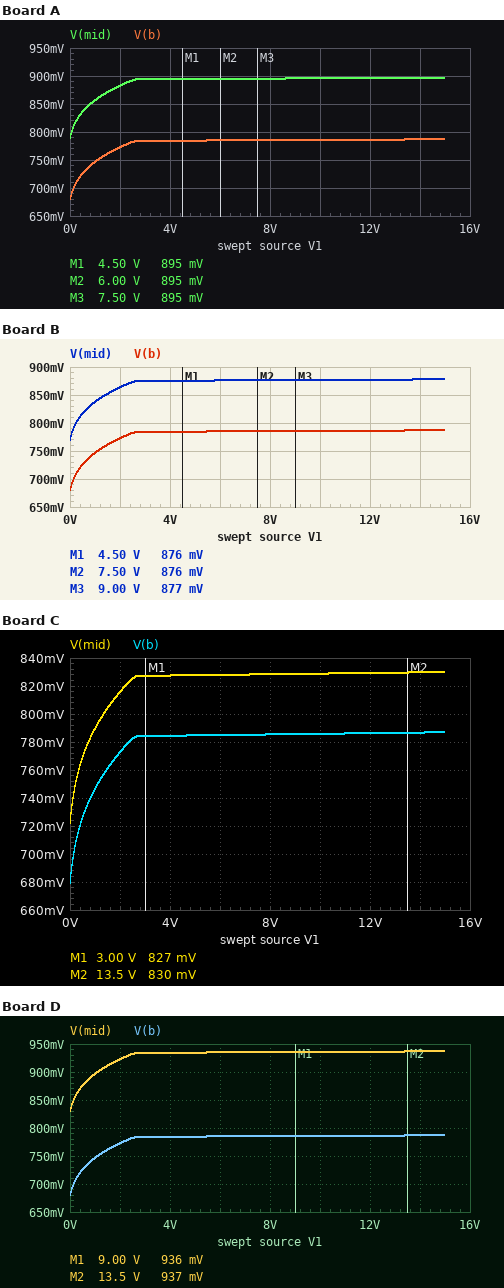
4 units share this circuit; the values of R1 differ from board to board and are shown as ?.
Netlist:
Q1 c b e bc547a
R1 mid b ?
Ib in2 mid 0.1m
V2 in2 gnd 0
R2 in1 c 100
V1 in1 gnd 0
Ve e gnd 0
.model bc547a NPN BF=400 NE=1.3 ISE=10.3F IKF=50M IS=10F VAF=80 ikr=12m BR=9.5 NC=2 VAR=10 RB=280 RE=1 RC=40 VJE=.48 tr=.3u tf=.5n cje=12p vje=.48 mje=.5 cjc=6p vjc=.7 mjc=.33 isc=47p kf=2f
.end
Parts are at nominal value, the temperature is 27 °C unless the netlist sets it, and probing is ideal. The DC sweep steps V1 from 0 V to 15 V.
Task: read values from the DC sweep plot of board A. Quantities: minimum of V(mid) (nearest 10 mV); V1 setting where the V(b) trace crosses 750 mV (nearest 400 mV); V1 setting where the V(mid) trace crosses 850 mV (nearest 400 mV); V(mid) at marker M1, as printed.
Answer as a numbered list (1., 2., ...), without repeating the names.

1. 790 mV
2. 1.2 V
3. 800 mV
4. 895 mV
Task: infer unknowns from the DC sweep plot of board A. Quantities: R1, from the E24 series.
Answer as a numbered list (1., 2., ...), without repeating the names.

1. 1.1 kΩ
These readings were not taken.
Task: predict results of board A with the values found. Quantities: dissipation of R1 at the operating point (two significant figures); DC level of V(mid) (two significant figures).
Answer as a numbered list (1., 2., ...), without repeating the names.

1. 11 µW
2. 790 mV
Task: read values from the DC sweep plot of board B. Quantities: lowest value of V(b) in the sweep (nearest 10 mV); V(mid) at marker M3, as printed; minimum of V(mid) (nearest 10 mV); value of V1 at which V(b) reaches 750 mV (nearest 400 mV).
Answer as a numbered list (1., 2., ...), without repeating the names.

1. 680 mV
2. 877 mV
3. 770 mV
4. 1.2 V
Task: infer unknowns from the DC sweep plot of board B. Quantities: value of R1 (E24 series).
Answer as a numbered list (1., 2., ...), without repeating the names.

1. 910 Ω
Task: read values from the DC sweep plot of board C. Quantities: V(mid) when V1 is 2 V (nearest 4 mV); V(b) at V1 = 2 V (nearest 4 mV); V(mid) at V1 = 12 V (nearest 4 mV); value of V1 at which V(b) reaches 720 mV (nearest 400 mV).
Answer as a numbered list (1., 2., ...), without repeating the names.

1. 816 mV
2. 772 mV
3. 828 mV
4. 400 mV
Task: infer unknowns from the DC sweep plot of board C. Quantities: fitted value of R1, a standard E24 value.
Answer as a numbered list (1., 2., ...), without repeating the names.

1. 430 Ω
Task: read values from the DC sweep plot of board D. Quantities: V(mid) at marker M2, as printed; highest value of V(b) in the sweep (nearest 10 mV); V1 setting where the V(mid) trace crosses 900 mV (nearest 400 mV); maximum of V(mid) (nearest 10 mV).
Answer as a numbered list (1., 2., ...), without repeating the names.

1. 937 mV
2. 790 mV
3. 1.2 V
4. 940 mV
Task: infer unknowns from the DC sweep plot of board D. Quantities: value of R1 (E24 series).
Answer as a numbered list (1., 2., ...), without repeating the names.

1. 1.5 kΩ
